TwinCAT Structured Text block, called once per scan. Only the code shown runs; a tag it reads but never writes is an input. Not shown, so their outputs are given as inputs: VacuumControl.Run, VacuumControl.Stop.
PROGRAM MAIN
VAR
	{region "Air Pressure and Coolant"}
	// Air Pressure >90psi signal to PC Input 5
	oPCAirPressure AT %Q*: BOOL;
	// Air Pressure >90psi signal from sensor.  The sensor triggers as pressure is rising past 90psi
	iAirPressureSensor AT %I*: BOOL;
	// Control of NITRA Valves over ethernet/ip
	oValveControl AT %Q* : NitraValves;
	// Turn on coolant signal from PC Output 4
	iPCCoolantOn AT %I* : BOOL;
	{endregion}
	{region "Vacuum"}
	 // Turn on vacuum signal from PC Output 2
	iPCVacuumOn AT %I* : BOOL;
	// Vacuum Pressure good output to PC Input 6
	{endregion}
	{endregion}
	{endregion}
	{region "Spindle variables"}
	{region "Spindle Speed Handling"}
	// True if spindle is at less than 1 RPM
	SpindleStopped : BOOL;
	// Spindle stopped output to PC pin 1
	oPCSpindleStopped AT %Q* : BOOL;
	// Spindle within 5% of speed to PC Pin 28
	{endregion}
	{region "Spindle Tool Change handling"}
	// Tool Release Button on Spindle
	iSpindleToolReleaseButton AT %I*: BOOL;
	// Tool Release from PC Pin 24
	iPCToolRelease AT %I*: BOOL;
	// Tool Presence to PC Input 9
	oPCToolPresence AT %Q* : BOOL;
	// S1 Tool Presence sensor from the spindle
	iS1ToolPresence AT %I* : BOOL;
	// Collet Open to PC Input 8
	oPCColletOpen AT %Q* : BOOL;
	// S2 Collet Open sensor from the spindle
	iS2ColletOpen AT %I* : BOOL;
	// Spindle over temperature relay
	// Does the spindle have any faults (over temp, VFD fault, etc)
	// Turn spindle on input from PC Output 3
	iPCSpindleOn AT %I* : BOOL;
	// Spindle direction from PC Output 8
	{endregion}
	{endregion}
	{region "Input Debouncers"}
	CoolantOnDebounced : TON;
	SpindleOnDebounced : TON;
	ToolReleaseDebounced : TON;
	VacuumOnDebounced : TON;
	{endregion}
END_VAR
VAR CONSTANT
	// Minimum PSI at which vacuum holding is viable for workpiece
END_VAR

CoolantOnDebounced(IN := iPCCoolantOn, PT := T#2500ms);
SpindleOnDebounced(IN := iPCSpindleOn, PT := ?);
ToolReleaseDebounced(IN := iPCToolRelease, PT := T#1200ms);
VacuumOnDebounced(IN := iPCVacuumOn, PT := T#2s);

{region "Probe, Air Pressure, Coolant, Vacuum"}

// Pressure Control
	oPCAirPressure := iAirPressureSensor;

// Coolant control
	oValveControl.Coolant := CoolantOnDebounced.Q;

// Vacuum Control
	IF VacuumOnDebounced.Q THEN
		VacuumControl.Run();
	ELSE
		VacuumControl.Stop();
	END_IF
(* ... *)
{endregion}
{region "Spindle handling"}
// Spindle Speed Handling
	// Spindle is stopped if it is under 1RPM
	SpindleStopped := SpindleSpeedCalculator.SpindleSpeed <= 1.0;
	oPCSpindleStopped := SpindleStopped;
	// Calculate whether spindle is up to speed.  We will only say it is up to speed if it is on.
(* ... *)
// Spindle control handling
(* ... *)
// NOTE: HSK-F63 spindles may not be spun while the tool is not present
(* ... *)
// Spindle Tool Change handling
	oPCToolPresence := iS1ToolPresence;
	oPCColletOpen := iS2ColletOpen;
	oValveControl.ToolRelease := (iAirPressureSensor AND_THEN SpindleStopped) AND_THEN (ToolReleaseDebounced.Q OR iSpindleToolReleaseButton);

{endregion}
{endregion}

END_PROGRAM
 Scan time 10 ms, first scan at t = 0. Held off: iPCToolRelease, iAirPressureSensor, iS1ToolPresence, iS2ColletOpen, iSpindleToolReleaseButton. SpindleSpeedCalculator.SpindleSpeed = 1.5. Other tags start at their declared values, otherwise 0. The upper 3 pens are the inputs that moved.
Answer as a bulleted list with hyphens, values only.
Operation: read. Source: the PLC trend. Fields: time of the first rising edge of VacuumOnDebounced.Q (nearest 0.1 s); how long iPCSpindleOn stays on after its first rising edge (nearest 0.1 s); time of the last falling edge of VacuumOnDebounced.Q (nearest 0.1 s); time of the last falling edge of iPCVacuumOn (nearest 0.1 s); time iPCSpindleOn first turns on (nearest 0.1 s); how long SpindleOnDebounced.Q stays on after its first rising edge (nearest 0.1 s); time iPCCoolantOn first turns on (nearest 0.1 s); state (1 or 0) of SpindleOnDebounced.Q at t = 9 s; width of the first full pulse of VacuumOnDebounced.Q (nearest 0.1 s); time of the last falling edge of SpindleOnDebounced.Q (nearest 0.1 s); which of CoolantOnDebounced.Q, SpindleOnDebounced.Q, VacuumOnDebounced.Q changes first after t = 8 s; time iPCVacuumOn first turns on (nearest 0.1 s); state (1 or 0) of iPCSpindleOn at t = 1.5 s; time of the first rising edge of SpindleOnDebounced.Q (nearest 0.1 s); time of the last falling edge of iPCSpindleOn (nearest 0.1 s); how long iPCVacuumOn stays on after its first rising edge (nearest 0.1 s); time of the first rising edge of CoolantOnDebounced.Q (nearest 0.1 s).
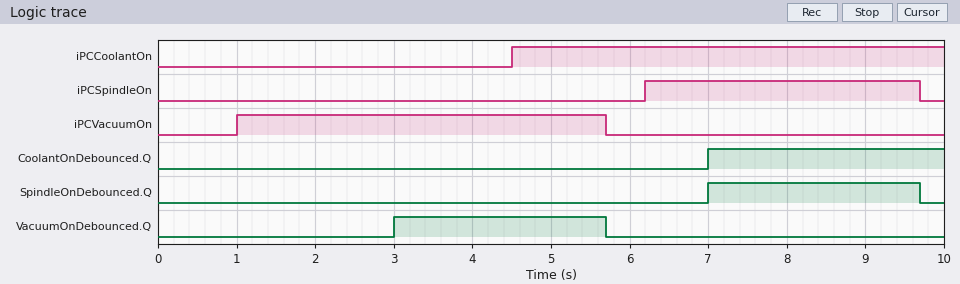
- 3.0 s
- 3.5 s
- 5.7 s
- 5.7 s
- 6.2 s
- 2.7 s
- 4.5 s
- 1
- 2.7 s
- 9.7 s
- SpindleOnDebounced.Q
- 1.0 s
- 0
- 7.0 s
- 9.7 s
- 4.7 s
- 7.0 s
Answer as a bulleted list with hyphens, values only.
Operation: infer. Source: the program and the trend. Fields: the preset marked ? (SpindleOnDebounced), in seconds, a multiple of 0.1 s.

- 0.8 s
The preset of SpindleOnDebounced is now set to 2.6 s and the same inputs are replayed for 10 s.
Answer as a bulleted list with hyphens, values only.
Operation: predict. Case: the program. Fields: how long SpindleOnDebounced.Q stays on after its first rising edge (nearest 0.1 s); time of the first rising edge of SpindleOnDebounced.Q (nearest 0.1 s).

- 0.9 s
- 8.8 s
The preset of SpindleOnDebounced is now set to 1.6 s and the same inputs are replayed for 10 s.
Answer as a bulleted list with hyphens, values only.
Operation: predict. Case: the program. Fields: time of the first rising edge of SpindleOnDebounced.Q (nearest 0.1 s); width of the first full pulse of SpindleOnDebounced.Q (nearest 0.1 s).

- 7.8 s
- 1.9 s
